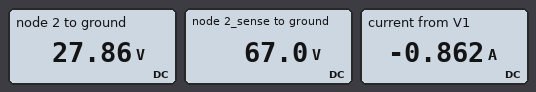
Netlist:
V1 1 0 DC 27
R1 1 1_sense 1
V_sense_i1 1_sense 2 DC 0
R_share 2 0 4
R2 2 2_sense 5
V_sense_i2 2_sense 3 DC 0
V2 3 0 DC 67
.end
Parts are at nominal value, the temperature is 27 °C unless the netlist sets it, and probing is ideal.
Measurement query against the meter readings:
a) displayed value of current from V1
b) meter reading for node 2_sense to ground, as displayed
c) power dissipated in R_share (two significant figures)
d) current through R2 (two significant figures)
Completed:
-0.862 A
67.0 V
190 W
7.8 A
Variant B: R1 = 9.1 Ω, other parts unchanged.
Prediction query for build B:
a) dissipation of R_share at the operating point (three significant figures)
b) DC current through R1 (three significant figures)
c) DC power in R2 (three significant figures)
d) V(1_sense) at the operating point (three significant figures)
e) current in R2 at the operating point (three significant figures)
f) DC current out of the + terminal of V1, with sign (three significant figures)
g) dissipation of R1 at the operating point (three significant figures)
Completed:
214 W
245 mA
285 W
29.2 V
7.55 A
-245 mA
548 mW
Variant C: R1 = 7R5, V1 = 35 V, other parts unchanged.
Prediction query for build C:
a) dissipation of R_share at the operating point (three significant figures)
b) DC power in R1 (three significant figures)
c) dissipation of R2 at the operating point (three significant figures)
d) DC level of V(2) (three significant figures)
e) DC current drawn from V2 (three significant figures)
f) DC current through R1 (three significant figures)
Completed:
240 W
2.16 W
260 W
31.0 V
7.21 A
537 mA
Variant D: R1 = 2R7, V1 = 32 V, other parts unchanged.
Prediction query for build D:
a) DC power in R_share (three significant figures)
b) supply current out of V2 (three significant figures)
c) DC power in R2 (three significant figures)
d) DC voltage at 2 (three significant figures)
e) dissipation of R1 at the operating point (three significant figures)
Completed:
237 W
7.24 A
262 W
30.8 V
550 mW
